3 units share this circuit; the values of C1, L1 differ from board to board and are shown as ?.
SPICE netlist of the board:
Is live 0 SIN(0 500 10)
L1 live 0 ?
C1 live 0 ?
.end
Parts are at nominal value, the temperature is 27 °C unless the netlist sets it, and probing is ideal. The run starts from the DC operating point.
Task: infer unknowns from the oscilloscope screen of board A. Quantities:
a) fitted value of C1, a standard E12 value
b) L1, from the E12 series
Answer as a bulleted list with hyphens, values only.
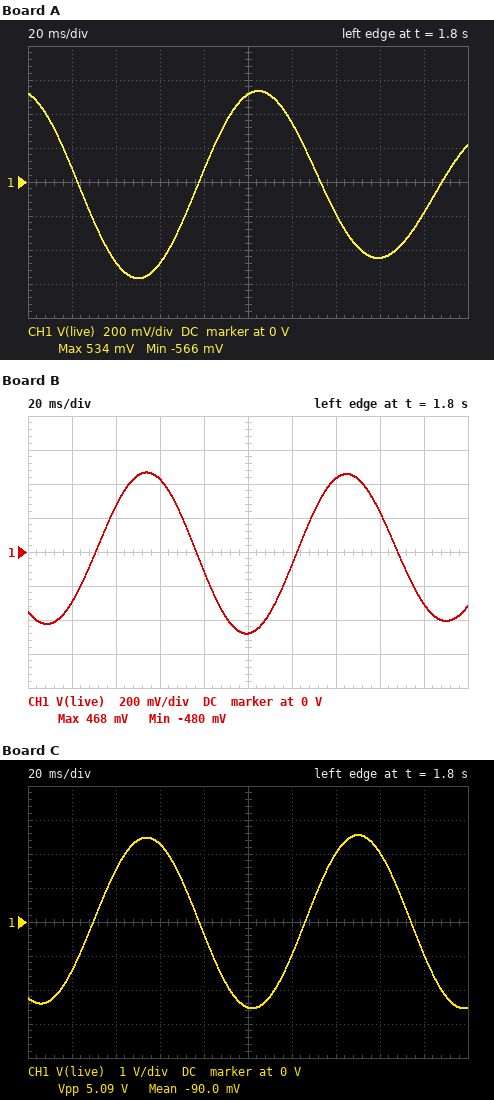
- 82 F
- 4.7 µH
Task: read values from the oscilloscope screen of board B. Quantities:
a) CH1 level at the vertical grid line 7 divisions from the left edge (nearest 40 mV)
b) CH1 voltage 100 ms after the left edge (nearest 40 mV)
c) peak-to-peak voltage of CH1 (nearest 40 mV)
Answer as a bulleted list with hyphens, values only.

- 440 mV
- -480 mV
- 960 mV
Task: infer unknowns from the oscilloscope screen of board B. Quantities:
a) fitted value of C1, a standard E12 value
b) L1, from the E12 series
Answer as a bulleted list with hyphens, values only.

- 82 F
- 2.2 µH
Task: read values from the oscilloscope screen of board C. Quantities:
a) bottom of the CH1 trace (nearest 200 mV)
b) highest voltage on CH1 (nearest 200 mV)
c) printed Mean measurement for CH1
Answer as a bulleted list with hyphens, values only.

- -2.6 V
- 2.6 V
- -90.0 mV
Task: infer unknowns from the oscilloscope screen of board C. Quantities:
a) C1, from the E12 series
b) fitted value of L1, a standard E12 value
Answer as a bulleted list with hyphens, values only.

- 39 F
- 5.6 µH
